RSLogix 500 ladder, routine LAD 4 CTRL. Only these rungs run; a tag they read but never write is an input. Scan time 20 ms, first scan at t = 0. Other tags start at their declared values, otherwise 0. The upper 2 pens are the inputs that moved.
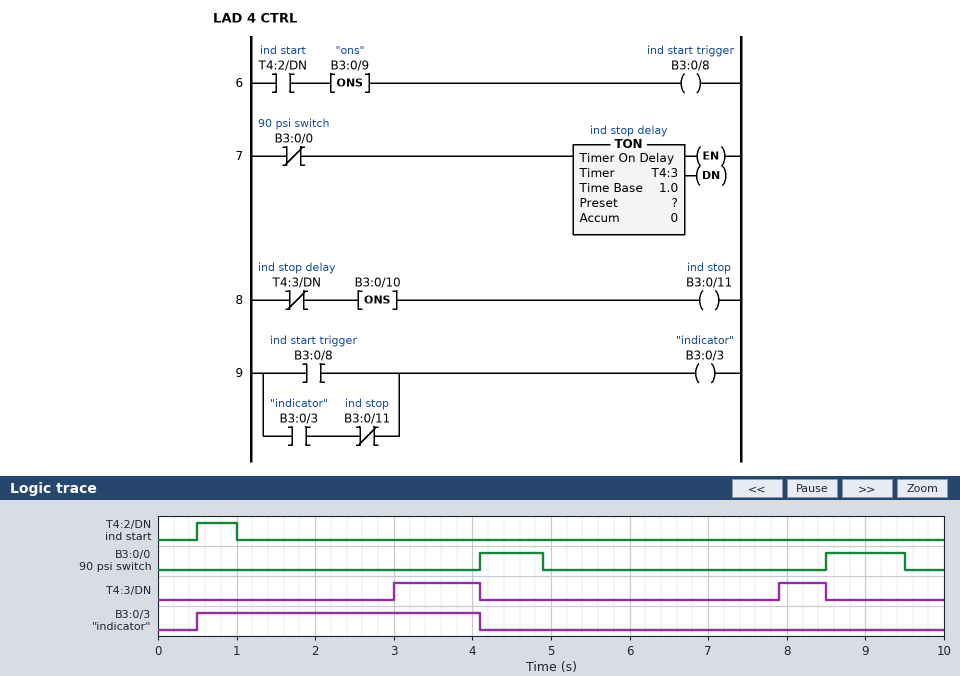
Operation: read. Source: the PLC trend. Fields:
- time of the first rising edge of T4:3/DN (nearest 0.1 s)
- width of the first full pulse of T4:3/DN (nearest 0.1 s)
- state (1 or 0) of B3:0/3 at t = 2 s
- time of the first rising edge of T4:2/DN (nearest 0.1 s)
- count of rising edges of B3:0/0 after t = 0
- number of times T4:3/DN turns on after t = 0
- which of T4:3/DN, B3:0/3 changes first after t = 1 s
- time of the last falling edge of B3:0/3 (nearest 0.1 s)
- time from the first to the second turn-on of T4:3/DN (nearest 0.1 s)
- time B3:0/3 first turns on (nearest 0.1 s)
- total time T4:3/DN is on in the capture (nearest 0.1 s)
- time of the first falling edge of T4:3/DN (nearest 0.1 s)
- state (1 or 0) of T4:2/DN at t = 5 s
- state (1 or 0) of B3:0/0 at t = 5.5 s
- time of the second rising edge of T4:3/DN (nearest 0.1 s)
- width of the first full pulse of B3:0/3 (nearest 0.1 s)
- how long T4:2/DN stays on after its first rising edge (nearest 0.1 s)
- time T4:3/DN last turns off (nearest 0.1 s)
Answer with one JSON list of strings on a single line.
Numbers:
["3.0 s", "1.1 s", "1", "0.5 s", "2", "2", "T4:3/DN", "4.1 s", "4.9 s", "0.5 s", "1.7 s", "4.1 s", "0", "0", "7.9 s", "3.6 s", "0.5 s", "8.5 s"]
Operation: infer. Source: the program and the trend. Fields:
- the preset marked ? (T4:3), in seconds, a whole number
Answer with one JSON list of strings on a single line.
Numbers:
["3 s"]
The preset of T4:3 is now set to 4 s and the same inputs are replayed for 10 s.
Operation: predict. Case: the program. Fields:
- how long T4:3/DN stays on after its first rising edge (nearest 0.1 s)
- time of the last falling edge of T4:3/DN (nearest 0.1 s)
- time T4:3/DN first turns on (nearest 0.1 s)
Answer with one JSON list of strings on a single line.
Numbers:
["0.1 s", "4.1 s", "4.0 s"]
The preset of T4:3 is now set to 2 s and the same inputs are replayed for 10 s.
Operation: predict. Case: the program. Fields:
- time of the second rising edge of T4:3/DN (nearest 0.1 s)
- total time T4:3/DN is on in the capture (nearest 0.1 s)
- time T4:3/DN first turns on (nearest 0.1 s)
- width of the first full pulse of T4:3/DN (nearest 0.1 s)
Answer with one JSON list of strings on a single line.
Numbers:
["6.9 s", "3.7 s", "2.0 s", "2.1 s"]
